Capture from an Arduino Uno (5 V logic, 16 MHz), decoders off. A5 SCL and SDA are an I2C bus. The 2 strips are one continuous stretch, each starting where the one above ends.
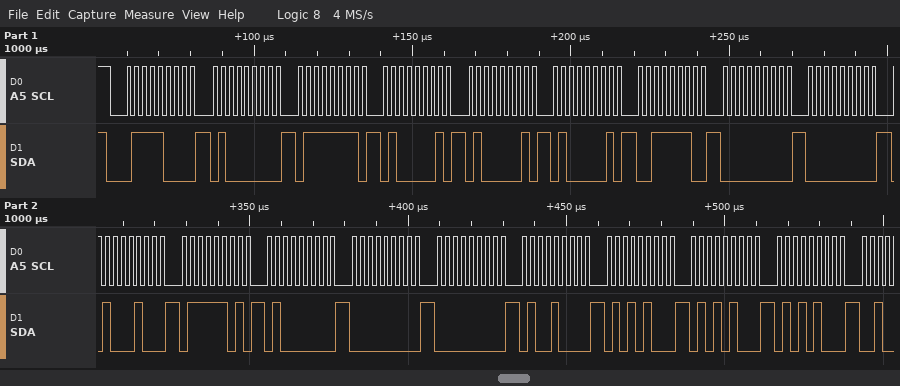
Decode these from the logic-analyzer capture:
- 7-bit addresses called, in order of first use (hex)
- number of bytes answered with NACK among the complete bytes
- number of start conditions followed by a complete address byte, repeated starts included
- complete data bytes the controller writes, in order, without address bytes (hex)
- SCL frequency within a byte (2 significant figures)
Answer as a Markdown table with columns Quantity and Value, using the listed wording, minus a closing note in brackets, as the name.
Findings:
| Quantity | Value |
|---|---|
| 7-bit addresses called, in order of first use | 0x3C |
| number of bytes answered with NACK among the complete bytes | 0 |
| number of start conditions followed by a complete address byte, repeated starts included | 1 |
| complete data bytes the controller writes, in order, without address bytes | 40 7F 41 41 41 3E 00 00 44 7D 40 00 00 48 54 54 54 |
| SCL frequency within a byte | 400 kHz |
